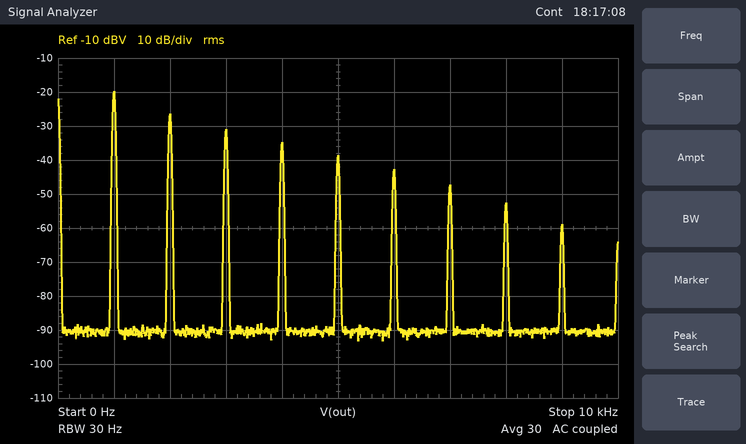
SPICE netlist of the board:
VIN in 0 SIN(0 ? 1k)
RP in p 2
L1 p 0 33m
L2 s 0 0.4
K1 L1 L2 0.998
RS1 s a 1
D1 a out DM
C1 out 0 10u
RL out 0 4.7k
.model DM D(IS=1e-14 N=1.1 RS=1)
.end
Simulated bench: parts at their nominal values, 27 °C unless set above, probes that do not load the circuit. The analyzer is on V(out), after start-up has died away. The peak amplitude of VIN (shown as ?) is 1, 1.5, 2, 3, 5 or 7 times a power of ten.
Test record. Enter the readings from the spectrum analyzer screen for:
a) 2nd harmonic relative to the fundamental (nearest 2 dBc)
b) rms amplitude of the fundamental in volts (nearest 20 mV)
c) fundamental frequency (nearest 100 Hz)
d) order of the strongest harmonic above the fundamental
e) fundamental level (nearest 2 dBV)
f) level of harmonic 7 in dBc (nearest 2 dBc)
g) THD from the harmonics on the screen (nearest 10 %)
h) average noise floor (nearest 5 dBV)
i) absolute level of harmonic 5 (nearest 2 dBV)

-6 dBc
100 mV
1.0 kHz
2
-20 dBV
-28 dBc
60 %
-90 dBV
-38 dBV
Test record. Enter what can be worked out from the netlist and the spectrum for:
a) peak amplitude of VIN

7 V
